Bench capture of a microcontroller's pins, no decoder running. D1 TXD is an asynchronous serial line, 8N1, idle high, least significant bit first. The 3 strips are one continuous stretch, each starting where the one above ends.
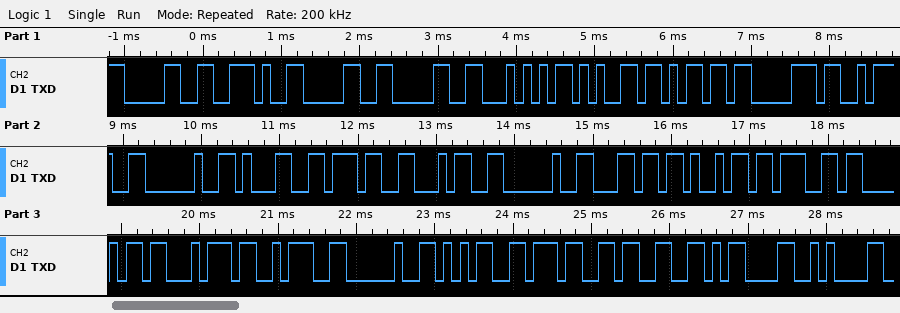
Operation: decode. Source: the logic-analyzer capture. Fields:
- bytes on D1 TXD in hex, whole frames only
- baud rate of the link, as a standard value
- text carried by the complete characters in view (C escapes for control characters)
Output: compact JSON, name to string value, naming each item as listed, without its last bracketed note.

{"bytes on D1 TXD in hex, whole frames only": "30 2E 30 30 54 65 6D 70 3A 20 31 37 34 20 6C 69 67 68 74 3A 20 35 37 33 0D 0A", "baud rate of the link, as a standard value": "9600 baud", "text carried by the complete characters in view": "\"0.00Temp: 174 light: 573\\r\\n\""}
